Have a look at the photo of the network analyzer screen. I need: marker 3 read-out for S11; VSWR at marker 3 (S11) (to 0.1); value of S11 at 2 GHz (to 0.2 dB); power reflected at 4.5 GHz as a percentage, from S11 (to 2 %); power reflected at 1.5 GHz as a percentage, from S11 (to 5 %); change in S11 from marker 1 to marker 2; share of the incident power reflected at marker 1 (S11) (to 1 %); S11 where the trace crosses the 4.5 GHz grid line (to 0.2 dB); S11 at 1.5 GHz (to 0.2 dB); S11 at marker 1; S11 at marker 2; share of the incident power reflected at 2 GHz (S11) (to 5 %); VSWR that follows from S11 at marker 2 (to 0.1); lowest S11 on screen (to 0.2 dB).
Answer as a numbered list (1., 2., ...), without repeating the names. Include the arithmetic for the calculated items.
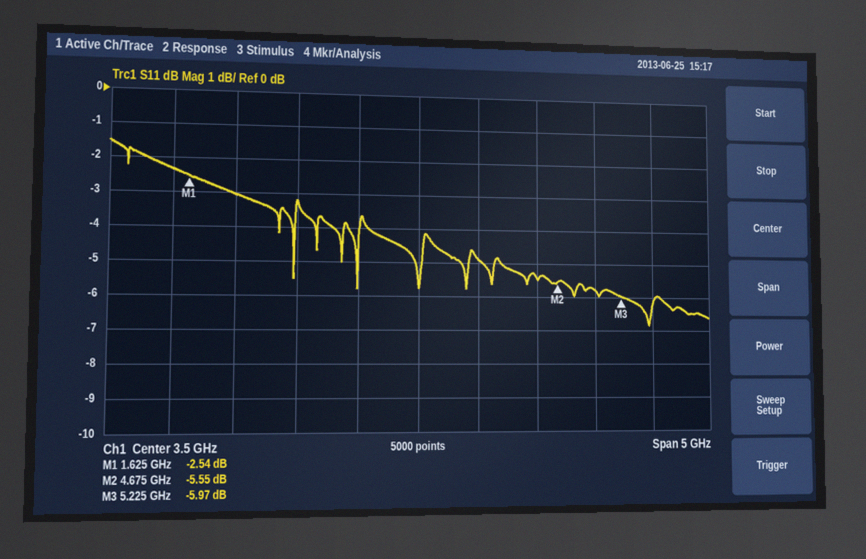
1. -5.97 dB
2. (1 + 0.5029)/(1 − 0.5029) ≈ 3.0
3. -3.0 dB
4. 10^(-5.4/10) ≈ 28.8 %, so 28 % to the nearest 2 %
5. 10^(-2.4/10) ≈ 57.5 %, so 60 % to the nearest 5 %
6. -5.55 − (-2.54) = -3.01 dB
7. 10^(-2.54/10) ≈ 56 %
8. -5.4 dB
9. -2.4 dB
10. -2.54 dB
11. -5.55 dB
12. 10^(-3/10) ≈ 50 %
13. (1 + 0.5278)/(1 − 0.5278) ≈ 3.2
14. -6.8 dB
